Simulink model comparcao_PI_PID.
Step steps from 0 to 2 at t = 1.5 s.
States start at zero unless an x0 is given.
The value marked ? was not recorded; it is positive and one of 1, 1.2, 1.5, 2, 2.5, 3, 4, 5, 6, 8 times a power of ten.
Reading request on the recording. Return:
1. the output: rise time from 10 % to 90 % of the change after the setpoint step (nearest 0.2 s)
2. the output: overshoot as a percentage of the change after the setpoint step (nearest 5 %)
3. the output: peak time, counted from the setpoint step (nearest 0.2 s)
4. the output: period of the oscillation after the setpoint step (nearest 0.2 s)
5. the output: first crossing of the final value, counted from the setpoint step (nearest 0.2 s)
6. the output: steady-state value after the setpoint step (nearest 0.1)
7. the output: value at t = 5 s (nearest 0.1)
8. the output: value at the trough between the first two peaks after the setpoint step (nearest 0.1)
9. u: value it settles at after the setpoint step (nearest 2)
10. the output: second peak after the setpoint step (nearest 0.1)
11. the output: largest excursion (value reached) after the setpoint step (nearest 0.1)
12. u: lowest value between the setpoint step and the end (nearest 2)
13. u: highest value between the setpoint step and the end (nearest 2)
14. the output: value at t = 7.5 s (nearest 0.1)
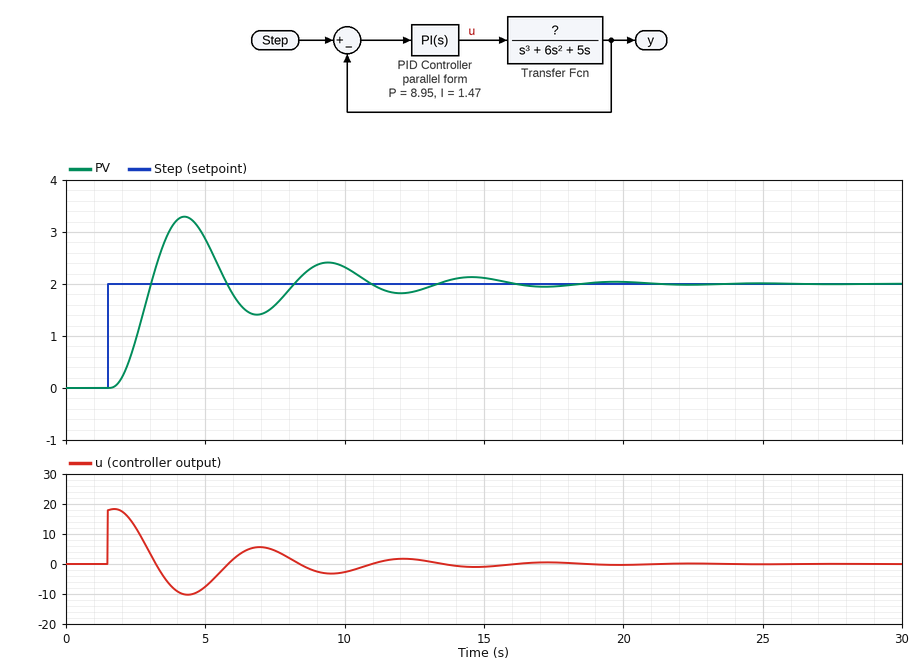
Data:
1.0 s
65 %
2.8 s
5.2 s
1.6 s
2.0
2.9
1.4
0
2.4
3.3
-10
18
1.6
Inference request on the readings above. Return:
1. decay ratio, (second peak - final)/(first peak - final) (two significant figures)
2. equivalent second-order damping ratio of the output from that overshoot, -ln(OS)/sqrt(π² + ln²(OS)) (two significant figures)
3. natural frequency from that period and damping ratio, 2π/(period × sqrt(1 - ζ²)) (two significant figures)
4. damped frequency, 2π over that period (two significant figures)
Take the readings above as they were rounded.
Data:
0.31
0.14
1.2 rad/s
1.2 rad/s
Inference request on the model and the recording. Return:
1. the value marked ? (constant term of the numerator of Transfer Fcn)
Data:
1
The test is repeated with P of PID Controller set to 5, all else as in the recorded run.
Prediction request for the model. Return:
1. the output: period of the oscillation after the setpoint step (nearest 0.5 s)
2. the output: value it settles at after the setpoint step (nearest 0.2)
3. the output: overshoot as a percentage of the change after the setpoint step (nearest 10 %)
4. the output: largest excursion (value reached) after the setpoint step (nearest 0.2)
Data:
7.5 s
2.0
70 %
3.4
